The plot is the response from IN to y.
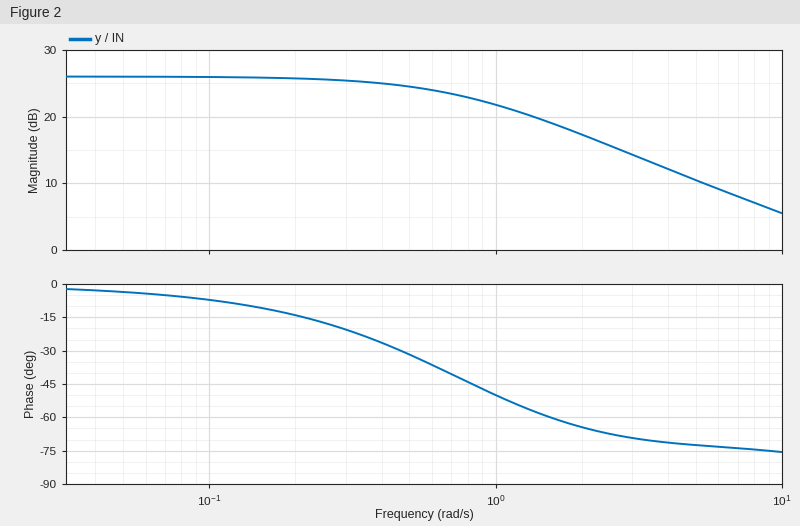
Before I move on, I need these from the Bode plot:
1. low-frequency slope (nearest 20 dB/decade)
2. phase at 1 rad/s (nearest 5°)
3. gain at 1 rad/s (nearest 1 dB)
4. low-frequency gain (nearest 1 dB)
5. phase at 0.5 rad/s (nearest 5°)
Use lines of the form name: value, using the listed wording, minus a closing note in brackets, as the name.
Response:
low-frequency slope: 0 dB/decade
phase at 1 rad/s: -50°
gain at 1 rad/s: 22 dB
low-frequency gain: 26 dB
phase at 0.5 rad/s: -30°
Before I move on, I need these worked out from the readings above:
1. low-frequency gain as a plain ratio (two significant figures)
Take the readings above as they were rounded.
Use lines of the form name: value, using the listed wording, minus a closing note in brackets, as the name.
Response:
low-frequency gain as a plain ratio: 20
